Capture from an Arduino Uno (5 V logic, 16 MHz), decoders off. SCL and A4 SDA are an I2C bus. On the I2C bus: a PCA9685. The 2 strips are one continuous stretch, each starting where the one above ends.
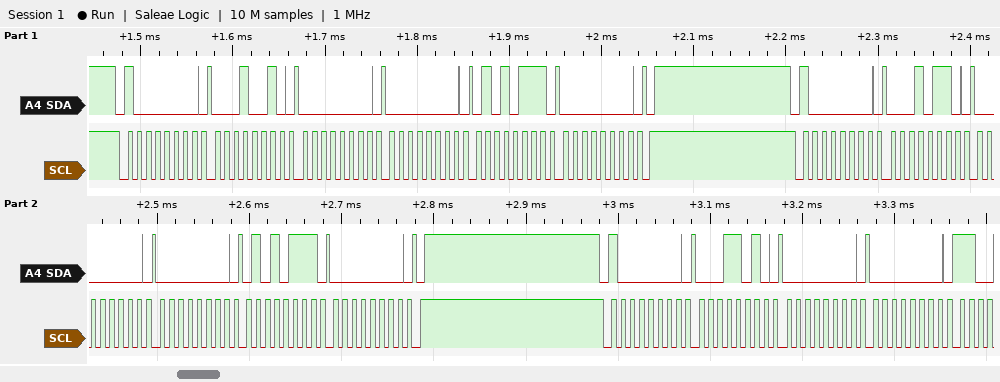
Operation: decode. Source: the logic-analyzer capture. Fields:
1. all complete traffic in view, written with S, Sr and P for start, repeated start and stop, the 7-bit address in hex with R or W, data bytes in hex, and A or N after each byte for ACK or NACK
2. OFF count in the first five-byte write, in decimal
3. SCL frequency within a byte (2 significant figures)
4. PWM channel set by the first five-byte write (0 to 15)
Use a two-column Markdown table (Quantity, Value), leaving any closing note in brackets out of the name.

| Quantity | Value |
|---|---|
| all complete traffic in view, written with S, Sr and P for start, repeated start and stop, the 7-bit address in hex with R or W, data bytes in hex, and A or N after each byte for ACK or NACK | S 40W A 12 A 00 A 00 A 57 A 00 A P S 40W A 16 A 00 A 00 A 57 A 00 A P S 40W A 1A A 00 A 00 A |
| OFF count in the first five-byte write, in decimal | 87 |
| SCL frequency within a byte | 100 kHz |
| PWM channel set by the first five-byte write | 3 |
